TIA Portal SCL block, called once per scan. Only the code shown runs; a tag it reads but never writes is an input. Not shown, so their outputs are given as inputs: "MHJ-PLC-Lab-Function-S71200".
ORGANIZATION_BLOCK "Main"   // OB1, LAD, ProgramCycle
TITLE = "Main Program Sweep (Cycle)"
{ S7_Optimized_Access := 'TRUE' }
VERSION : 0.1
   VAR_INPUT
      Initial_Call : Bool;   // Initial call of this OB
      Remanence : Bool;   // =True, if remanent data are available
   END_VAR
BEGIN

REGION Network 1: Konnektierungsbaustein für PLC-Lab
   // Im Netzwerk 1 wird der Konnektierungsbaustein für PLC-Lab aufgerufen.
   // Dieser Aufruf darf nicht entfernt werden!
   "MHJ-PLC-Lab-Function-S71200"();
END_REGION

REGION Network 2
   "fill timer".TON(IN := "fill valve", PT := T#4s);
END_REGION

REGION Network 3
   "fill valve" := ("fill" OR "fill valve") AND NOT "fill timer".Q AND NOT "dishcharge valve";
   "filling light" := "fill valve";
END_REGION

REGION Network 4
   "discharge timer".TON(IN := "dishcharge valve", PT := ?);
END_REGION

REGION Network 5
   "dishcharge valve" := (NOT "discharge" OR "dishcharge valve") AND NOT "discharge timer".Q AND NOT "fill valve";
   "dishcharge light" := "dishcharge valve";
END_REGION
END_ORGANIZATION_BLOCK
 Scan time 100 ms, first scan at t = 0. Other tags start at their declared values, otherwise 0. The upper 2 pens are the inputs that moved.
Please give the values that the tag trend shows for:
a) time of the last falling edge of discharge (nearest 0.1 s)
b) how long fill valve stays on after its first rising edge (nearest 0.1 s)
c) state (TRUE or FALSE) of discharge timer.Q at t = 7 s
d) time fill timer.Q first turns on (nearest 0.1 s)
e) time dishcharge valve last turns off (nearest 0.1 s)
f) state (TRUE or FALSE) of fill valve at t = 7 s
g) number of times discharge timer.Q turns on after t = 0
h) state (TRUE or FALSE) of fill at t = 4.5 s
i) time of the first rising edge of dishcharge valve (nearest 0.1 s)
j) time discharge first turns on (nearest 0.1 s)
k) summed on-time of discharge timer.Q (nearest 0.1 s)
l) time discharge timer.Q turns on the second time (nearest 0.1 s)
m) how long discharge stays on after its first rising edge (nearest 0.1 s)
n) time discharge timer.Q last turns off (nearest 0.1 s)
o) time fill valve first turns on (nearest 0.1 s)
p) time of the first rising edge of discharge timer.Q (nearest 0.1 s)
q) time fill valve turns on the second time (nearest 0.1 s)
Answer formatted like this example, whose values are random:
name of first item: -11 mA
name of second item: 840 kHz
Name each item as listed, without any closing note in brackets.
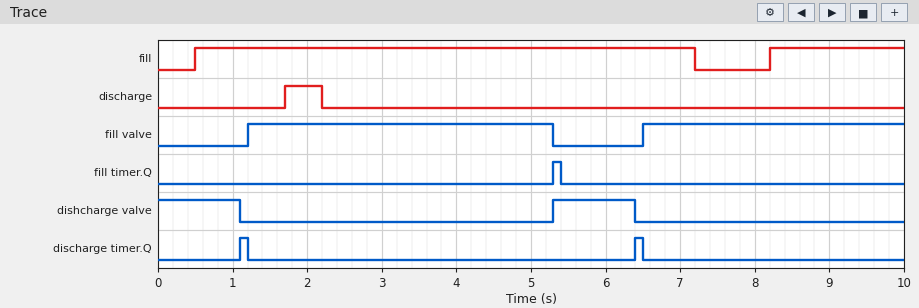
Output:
time of the last falling edge of discharge: 2.2 s
how long fill valve stays on after its first rising edge: 4.1 s
state (TRUE or FALSE) of discharge timer.Q at t = 7 s: FALSE
time fill timer.Q first turns on: 5.3 s
time dishcharge valve last turns off: 6.4 s
state (TRUE or FALSE) of fill valve at t = 7 s: TRUE
number of times discharge timer.Q turns on after t = 0: 2
state (TRUE or FALSE) of fill at t = 4.5 s: TRUE
time of the first rising edge of dishcharge valve: 5.3 s
time discharge first turns on: 1.7 s
summed on-time of discharge timer.Q: 0.2 s
time discharge timer.Q turns on the second time: 6.4 s
how long discharge stays on after its first rising edge: 0.5 s
time discharge timer.Q last turns off: 6.5 s
time fill valve first turns on: 1.2 s
time of the first rising edge of discharge timer.Q: 1.1 s
time fill valve turns on the second time: 6.5 s
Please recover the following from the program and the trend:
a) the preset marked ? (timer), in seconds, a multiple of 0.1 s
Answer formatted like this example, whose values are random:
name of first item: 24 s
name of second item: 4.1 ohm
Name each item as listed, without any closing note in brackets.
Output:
the preset marked ? (timer), in seconds, a multiple of 0.1 s: 1.0 s
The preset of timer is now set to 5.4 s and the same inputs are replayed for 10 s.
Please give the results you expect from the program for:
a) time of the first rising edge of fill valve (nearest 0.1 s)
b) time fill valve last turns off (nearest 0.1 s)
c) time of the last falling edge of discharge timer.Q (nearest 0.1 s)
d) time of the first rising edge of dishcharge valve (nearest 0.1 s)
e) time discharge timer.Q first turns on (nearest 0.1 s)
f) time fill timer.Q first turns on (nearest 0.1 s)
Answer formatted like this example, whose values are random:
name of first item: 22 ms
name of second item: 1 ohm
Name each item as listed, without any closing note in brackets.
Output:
time of the first rising edge of fill valve: 5.6 s
time fill valve last turns off: 9.7 s
time of the last falling edge of discharge timer.Q: 5.6 s
time of the first rising edge of dishcharge valve: 9.7 s
time discharge timer.Q first turns on: 5.5 s
time fill timer.Q first turns on: 9.7 s
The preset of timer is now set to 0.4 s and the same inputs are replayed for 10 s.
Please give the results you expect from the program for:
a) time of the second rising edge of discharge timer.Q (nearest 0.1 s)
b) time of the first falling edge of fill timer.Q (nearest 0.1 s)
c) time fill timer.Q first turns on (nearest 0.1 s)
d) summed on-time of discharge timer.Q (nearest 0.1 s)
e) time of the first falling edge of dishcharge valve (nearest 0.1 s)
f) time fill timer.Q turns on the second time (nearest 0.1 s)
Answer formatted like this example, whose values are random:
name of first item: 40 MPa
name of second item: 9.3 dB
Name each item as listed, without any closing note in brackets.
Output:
time of the second rising edge of discharge timer.Q: 5.2 s
time of the first falling edge of fill timer.Q: 4.8 s
time fill timer.Q first turns on: 4.7 s
summed on-time of discharge timer.Q: 0.3 s
time of the first falling edge of dishcharge valve: 0.5 s
time fill timer.Q turns on the second time: 9.4 s
